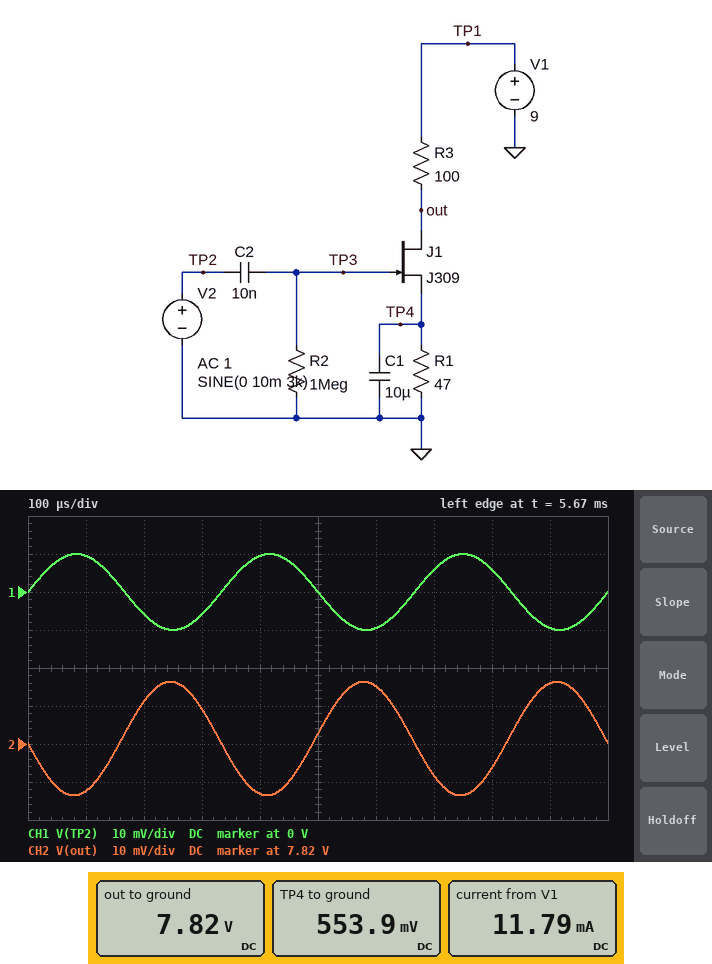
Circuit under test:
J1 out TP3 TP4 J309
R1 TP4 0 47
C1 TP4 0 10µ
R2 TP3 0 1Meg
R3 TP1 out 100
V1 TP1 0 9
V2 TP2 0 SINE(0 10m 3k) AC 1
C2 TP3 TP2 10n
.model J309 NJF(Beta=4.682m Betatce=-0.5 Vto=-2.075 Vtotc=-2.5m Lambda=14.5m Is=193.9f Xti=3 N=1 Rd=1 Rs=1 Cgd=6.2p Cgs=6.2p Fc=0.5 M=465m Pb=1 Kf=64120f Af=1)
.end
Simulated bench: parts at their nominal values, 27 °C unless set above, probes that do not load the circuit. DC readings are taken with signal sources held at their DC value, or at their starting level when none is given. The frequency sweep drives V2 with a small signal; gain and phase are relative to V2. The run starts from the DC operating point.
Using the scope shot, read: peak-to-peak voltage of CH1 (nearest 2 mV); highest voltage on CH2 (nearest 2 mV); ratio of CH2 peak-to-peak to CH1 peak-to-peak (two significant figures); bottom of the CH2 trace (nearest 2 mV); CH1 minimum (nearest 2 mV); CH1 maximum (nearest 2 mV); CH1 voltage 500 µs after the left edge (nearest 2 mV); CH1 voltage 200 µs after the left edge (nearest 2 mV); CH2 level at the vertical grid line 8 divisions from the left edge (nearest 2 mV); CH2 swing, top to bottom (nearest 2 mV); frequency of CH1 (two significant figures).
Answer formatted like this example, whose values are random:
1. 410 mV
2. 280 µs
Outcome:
1. 20 mV
2. 7.836 V
3. 1.5
4. 7.806 V
5. -10 mV
6. 10 mV
7. 0 V
8. -6 mV
9. 7.814 V
10. 30 mV
11. 3.0 kHz
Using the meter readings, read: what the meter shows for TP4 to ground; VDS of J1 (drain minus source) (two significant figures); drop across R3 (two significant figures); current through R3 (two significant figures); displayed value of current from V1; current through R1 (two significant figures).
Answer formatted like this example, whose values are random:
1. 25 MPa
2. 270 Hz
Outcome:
1. 553.9 mV
2. 7.3 V
3. 1.2 V
4. 12 mA
5. 11.79 mA
6. 12 mA
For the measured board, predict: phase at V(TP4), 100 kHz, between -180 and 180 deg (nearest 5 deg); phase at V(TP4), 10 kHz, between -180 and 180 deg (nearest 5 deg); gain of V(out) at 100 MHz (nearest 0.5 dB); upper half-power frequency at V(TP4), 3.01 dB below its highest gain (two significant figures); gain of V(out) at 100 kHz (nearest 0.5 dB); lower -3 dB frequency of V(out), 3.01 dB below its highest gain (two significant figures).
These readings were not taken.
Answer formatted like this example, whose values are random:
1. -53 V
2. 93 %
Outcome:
1. -90 deg
2. -85 deg
3. 3.5 dB
4. 610 Hz
5. 3.5 dB
6. 330 Hz
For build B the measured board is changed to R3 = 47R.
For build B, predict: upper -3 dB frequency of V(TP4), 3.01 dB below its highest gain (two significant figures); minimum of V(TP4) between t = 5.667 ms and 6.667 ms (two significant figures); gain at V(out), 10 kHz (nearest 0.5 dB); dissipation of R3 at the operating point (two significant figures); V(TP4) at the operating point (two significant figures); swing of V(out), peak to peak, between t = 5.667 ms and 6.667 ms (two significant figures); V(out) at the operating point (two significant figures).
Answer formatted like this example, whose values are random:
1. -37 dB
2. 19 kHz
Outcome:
1. 620 Hz
2. 560 mV
3. -3.0 dB
4. 6.6 mW
5. 560 mV
6. 14 mV
7. 8.4 V
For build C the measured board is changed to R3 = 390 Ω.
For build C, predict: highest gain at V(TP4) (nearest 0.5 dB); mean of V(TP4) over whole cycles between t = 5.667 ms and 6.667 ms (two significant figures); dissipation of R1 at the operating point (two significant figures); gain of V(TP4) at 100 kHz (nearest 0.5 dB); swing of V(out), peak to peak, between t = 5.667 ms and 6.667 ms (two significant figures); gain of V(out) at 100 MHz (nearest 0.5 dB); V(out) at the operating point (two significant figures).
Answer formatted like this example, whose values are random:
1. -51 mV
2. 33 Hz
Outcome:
1. -8.5 dB
2. 540 mV
3. 6.2 mW
4. -53.0 dB
5. 110 mV
6. 13.5 dB
7. 4.5 V
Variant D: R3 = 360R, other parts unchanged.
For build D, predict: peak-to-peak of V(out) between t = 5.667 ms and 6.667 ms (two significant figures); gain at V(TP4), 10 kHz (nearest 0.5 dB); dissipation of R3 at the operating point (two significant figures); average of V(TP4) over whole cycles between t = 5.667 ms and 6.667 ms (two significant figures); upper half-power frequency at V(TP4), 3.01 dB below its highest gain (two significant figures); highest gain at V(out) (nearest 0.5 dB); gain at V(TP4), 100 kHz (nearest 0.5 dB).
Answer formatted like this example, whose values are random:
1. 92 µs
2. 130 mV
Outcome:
1. 100 mV
2. -33.0 dB
3. 48 mW
4. 540 mV
5. 600 Hz
6. 14.0 dB
7. -53.0 dB
